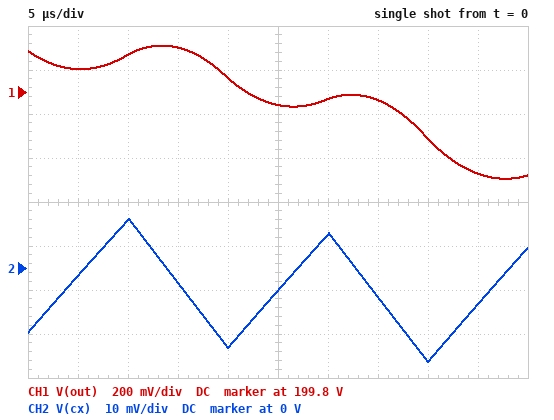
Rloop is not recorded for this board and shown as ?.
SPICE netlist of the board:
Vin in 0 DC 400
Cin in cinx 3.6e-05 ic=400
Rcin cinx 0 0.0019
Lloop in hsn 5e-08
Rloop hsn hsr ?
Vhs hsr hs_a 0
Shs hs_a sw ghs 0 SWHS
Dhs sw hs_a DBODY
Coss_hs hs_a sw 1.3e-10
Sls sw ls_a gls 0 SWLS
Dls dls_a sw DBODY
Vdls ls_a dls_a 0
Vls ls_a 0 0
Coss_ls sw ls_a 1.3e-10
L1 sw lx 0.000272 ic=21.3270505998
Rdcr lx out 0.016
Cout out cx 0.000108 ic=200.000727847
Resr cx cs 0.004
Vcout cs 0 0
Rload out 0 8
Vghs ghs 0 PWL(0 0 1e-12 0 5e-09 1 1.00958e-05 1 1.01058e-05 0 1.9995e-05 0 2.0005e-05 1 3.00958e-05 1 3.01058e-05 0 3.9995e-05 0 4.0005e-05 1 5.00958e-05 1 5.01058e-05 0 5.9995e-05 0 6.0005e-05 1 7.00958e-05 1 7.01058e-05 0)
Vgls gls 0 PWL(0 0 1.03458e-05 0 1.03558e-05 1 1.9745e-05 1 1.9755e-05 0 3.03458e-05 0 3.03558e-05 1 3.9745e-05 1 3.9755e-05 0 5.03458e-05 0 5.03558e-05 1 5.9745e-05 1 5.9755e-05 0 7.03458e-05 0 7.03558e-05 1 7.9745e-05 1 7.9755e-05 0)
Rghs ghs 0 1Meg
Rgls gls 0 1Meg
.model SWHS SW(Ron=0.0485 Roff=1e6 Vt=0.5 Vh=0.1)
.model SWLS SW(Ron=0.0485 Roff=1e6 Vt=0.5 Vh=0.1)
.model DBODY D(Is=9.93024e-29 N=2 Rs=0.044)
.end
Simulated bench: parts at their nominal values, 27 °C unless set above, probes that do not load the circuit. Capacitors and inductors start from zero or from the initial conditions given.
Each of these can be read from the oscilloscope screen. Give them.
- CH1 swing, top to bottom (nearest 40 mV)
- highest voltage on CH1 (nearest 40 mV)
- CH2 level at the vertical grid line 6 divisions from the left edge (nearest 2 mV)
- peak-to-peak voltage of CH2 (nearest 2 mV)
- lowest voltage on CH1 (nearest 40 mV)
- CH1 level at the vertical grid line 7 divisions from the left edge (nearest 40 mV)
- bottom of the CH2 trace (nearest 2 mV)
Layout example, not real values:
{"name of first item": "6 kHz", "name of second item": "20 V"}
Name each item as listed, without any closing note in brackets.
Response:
{"CH1 swing, top to bottom": "600 mV", "highest voltage on CH1": "200.00 V", "CH2 level at the vertical grid line 6 divisions from the left edge": "8 mV", "peak-to-peak voltage of CH2": "32 mV", "lowest voltage on CH1": "199.40 V", "CH1 level at the vertical grid line 7 divisions from the left edge": "199.76 V", "bottom of the CH2 trace": "-22 mV"}
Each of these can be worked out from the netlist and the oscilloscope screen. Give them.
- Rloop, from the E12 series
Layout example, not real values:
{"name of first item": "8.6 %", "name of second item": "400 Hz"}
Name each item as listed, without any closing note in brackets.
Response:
{"Rloop, from the E12 series": "1 Ω"}
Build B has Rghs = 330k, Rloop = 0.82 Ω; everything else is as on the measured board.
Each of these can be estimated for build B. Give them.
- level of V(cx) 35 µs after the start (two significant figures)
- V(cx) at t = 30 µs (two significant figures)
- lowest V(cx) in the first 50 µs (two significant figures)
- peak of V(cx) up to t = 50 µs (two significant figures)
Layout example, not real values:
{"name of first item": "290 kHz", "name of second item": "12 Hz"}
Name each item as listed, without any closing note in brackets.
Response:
{"level of V(cx) 35 µs after the start": "-5.4 mV", "V(cx) at t = 30 µs": "8.8 mV", "lowest V(cx) in the first 50 µs": "-20 mV", "peak of V(cx) up to t = 50 µs": "12 mV"}
